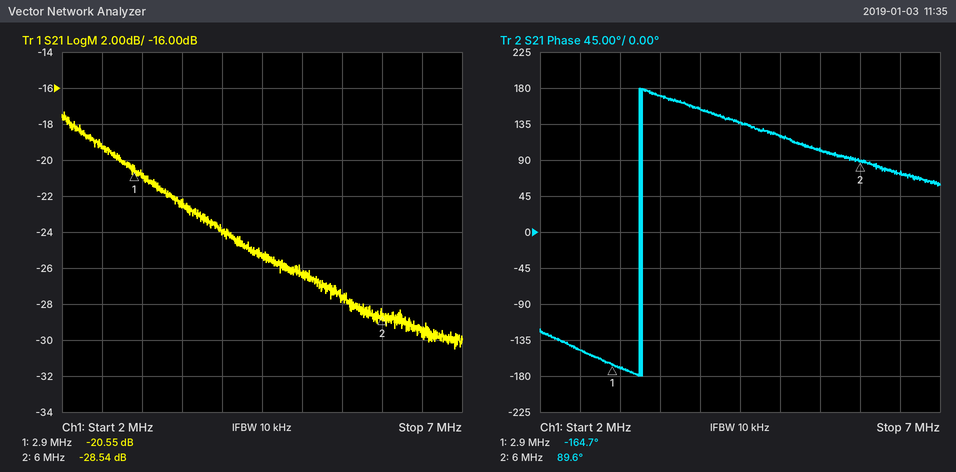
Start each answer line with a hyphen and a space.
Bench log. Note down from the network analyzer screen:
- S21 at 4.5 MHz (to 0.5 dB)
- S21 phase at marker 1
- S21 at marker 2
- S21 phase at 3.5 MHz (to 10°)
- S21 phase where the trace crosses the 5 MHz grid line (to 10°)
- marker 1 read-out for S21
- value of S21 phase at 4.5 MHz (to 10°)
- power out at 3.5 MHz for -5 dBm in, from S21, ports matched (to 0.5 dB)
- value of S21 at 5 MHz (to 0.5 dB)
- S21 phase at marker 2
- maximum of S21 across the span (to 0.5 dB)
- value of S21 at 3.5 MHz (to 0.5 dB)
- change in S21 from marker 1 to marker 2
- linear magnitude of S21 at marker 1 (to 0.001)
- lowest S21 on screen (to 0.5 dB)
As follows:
- -25.5 dB
- -164.7°
- -28.54 dB
- 170°
- 120°
- -20.55 dB
- 140°
- -27.5 dBm
- -26.5 dB
- 89.6°
- -17.5 dB
- -22.5 dB
- -7.99 dB
- 0.094
- -30.5 dB
